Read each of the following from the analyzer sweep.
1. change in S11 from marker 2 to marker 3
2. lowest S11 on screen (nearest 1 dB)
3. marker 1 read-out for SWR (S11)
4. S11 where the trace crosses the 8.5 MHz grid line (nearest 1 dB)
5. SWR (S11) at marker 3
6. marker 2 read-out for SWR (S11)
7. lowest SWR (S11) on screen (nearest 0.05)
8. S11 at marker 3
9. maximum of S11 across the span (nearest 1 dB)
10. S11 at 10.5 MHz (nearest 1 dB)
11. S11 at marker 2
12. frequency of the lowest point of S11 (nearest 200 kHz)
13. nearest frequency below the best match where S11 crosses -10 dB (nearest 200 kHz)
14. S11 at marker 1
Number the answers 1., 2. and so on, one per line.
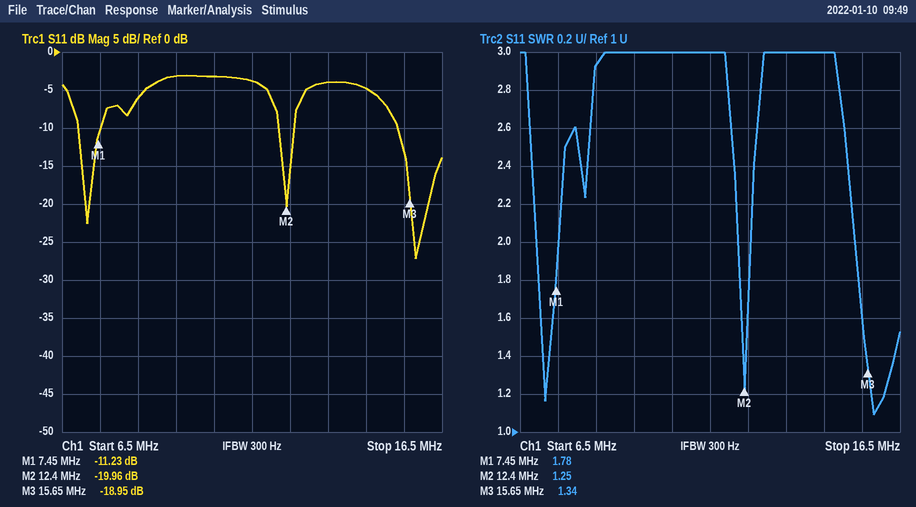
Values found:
1. 1.01 dB
2. -27 dB
3. 1.78
4. -6 dB
5. 1.34
6. 1.25
7. 1.10
8. -18.95 dB
9. -3 dB
10. -3 dB
11. -19.96 dB
12. 15.8 MHz
13. 15.4 MHz
14. -11.23 dB
